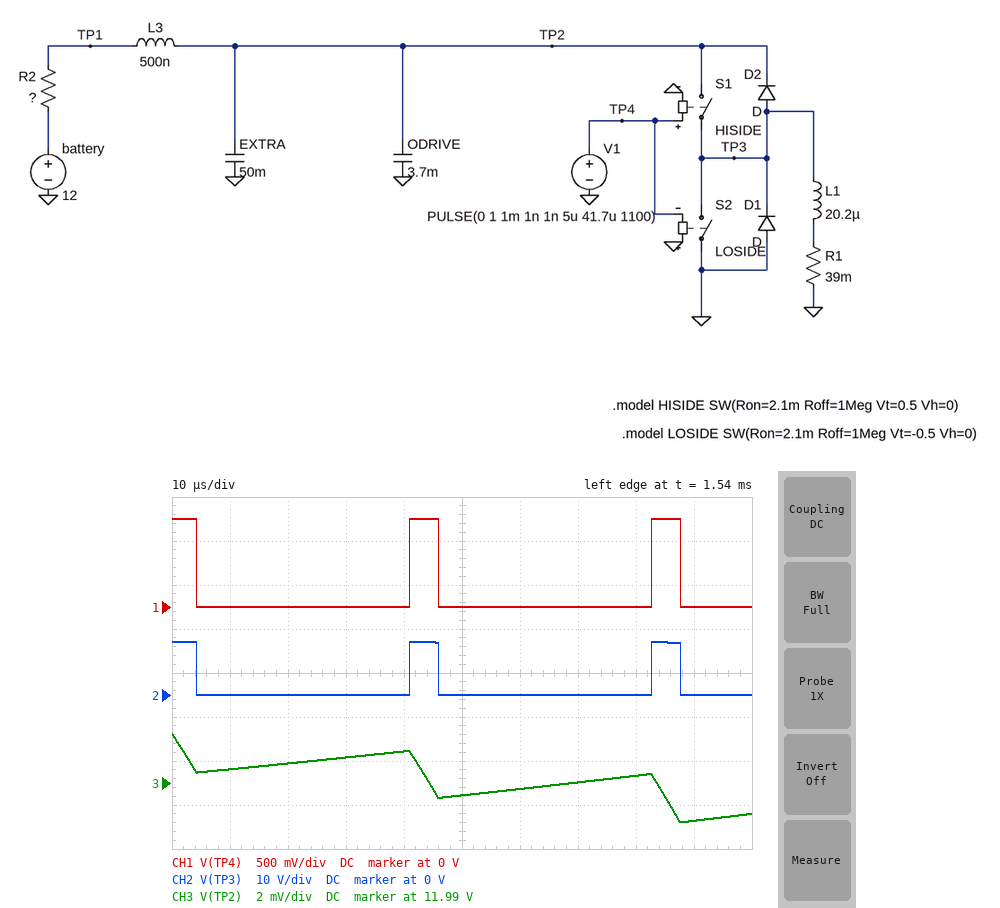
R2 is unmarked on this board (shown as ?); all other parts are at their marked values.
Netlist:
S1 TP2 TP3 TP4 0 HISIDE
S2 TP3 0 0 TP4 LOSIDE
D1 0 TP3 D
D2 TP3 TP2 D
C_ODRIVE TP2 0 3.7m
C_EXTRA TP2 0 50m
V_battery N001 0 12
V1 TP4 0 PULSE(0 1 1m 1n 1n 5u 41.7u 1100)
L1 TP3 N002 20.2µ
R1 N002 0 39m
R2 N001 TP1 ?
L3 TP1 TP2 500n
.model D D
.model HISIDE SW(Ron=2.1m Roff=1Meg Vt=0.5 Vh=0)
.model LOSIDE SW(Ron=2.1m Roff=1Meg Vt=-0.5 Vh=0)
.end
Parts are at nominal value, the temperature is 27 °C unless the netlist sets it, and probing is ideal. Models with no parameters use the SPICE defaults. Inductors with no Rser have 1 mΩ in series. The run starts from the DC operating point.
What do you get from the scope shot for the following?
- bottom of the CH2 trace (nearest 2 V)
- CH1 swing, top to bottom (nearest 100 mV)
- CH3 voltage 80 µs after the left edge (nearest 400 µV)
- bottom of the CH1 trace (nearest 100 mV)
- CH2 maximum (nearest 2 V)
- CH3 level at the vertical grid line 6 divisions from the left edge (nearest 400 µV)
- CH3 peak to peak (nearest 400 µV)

0 V
1.0 V
11.9864 V
0 V
12 V
11.9856 V
4.0 mV
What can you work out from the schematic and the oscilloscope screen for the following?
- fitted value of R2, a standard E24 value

6.8 mΩ
